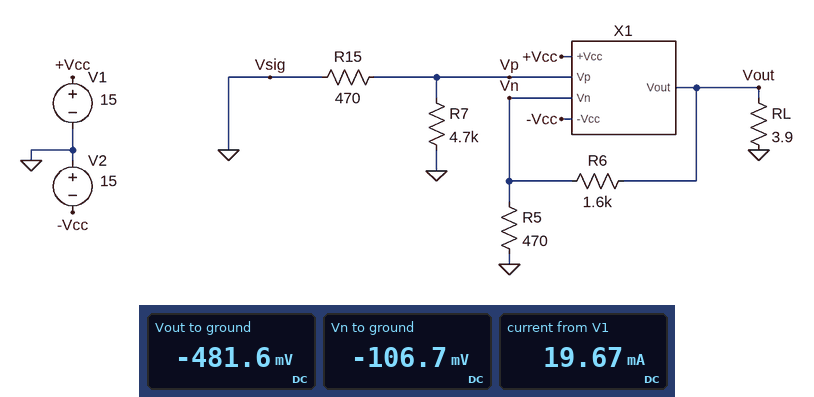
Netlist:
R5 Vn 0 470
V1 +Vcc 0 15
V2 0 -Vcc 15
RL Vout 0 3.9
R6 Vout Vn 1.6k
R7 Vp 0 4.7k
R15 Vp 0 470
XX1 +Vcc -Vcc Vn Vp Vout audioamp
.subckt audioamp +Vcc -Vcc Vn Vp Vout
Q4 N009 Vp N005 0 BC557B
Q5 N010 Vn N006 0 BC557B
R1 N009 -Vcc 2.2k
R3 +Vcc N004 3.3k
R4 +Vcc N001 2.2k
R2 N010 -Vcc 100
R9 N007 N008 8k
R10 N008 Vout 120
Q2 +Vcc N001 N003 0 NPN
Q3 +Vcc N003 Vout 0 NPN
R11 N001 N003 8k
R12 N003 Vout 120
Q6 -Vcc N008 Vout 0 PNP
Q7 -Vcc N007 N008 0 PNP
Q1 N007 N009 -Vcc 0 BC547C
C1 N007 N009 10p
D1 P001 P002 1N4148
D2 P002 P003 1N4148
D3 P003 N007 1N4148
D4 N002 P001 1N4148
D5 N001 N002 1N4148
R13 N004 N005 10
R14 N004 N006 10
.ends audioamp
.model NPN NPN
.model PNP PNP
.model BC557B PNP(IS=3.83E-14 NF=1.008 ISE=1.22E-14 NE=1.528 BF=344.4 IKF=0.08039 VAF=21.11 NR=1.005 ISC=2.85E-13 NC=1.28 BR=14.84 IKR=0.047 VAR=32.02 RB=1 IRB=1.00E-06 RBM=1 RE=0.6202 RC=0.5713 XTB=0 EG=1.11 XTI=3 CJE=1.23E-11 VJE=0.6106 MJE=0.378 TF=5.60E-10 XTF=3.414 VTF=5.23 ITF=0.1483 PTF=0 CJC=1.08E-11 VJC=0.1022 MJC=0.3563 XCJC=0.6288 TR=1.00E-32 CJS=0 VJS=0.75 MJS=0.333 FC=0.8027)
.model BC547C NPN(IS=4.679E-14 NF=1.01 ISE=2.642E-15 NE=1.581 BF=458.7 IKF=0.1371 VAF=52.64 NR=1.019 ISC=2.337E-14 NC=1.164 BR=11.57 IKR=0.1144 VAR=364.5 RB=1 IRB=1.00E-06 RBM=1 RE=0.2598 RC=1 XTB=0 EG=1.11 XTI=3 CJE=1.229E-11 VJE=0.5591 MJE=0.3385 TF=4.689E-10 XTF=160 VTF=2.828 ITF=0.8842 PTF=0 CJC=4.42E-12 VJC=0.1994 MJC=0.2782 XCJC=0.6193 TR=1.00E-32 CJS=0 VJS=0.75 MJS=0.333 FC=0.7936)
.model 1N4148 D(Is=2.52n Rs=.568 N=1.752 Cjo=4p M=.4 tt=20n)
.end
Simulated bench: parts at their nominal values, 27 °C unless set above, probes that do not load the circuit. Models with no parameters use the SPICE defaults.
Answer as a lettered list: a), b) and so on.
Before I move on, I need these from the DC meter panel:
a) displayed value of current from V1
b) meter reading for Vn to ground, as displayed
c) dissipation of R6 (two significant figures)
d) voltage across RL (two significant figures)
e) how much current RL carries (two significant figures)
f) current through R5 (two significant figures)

a) 19.67 mA
b) -106.7 mV
c) 88 µW
d) 480 mV
e) 120 mA
f) 230 µA
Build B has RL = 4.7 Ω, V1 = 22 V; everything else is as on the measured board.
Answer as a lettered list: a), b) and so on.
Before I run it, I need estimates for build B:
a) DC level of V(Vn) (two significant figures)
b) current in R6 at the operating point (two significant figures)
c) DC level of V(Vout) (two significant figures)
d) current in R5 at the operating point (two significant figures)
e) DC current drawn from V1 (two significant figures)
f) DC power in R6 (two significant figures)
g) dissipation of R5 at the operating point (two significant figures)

a) -140 mV
b) 310 µA
c) -630 mV
d) 300 µA
e) 90 mA
f) 150 µW
g) 41 µW
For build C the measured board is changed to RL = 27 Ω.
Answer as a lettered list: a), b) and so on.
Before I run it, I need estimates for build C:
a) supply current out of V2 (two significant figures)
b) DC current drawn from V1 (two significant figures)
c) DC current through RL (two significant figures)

a) 47 mA
b) 29 mA
c) 18 mA
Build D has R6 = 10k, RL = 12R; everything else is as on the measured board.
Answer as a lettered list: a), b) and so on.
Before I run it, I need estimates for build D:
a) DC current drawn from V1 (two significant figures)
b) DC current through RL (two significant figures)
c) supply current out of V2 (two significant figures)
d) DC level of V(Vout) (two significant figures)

a) 23 mA
b) 200 mA
c) 230 mA
d) -2.4 V
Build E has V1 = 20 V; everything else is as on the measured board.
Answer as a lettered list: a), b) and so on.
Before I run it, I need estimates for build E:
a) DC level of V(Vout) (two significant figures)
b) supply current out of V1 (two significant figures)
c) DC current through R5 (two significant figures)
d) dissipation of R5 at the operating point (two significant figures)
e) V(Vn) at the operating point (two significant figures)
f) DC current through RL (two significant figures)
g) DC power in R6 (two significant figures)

a) -590 mV
b) 51 mA
c) 280 µA
d) 36 µW
e) -130 mV
f) 150 mA
g) 130 µW
